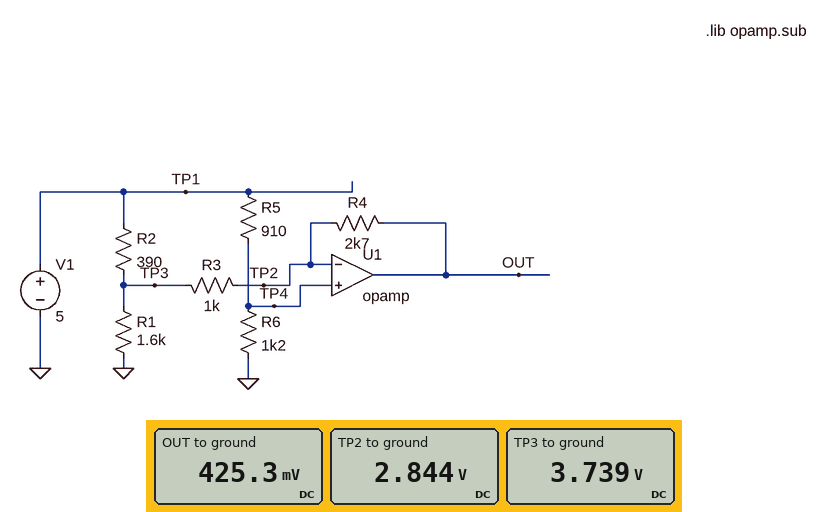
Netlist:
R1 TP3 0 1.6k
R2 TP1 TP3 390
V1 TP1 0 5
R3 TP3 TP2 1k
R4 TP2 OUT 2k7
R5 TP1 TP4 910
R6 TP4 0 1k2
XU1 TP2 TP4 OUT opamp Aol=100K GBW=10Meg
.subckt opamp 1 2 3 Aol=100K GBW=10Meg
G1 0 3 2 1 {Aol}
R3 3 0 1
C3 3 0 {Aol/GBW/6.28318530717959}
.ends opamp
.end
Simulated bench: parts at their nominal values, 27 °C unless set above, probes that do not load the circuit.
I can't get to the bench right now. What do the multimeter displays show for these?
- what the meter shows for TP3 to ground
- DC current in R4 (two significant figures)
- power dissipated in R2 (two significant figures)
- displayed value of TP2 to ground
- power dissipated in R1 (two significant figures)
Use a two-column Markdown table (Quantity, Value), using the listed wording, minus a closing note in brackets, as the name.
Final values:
| Quantity | Value |
|---|---|
| what the meter shows for TP3 to ground | 3.739 V |
| DC current in R4 | 900 µA |
| power dissipated in R2 | 4.1 mW |
| displayed value of TP2 to ground | 2.844 V |
| power dissipated in R1 | 8.7 mW |
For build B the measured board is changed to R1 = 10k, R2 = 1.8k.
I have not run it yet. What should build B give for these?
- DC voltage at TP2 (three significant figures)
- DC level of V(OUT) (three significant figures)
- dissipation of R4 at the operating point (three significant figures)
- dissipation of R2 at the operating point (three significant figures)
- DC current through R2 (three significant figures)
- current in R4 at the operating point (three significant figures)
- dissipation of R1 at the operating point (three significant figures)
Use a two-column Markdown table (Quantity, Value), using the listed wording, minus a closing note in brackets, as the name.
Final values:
| Quantity | Value |
|---|---|
| DC voltage at TP2 | 2.84 V |
| DC level of V(OUT) | 1.35 V |
| dissipation of R4 at the operating point | 822 µW |
| dissipation of R2 at the operating point | 1.43 mW |
| DC current through R2 | 891 µA |
| current in R4 at the operating point | 552 µA |
| dissipation of R1 at the operating point | 1.15 mW |
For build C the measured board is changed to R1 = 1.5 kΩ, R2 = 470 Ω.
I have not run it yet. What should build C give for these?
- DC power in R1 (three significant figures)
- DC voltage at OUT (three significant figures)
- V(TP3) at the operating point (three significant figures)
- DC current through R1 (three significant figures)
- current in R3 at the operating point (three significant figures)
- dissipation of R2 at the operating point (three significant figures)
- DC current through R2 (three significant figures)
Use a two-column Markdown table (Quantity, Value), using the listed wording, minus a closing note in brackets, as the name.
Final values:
| Quantity | Value |
|---|---|
| DC power in R1 | 8.42 mW |
| DC voltage at OUT | 928 mV |
| V(TP3) at the operating point | 3.55 V |
| DC current through R1 | 2.37 mA |
| current in R3 at the operating point | 710 µA |
| dissipation of R2 at the operating point | 4.45 mW |
| DC current through R2 | 3.08 mA |
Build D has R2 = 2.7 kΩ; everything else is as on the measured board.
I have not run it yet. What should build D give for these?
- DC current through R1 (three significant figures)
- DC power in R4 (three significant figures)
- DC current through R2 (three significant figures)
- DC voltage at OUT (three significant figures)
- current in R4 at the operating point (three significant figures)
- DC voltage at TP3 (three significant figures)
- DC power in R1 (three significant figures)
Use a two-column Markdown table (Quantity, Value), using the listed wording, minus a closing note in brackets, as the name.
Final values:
| Quantity | Value |
|---|---|
| DC current through R1 | 1.47 mA |
| DC power in R4 | 649 µW |
| DC current through R2 | 980 µA |
| DC voltage at OUT | 4.17 V |
| current in R4 at the operating point | 490 µA |
| DC voltage at TP3 | 2.35 V |
| DC power in R1 | 3.46 mW |
